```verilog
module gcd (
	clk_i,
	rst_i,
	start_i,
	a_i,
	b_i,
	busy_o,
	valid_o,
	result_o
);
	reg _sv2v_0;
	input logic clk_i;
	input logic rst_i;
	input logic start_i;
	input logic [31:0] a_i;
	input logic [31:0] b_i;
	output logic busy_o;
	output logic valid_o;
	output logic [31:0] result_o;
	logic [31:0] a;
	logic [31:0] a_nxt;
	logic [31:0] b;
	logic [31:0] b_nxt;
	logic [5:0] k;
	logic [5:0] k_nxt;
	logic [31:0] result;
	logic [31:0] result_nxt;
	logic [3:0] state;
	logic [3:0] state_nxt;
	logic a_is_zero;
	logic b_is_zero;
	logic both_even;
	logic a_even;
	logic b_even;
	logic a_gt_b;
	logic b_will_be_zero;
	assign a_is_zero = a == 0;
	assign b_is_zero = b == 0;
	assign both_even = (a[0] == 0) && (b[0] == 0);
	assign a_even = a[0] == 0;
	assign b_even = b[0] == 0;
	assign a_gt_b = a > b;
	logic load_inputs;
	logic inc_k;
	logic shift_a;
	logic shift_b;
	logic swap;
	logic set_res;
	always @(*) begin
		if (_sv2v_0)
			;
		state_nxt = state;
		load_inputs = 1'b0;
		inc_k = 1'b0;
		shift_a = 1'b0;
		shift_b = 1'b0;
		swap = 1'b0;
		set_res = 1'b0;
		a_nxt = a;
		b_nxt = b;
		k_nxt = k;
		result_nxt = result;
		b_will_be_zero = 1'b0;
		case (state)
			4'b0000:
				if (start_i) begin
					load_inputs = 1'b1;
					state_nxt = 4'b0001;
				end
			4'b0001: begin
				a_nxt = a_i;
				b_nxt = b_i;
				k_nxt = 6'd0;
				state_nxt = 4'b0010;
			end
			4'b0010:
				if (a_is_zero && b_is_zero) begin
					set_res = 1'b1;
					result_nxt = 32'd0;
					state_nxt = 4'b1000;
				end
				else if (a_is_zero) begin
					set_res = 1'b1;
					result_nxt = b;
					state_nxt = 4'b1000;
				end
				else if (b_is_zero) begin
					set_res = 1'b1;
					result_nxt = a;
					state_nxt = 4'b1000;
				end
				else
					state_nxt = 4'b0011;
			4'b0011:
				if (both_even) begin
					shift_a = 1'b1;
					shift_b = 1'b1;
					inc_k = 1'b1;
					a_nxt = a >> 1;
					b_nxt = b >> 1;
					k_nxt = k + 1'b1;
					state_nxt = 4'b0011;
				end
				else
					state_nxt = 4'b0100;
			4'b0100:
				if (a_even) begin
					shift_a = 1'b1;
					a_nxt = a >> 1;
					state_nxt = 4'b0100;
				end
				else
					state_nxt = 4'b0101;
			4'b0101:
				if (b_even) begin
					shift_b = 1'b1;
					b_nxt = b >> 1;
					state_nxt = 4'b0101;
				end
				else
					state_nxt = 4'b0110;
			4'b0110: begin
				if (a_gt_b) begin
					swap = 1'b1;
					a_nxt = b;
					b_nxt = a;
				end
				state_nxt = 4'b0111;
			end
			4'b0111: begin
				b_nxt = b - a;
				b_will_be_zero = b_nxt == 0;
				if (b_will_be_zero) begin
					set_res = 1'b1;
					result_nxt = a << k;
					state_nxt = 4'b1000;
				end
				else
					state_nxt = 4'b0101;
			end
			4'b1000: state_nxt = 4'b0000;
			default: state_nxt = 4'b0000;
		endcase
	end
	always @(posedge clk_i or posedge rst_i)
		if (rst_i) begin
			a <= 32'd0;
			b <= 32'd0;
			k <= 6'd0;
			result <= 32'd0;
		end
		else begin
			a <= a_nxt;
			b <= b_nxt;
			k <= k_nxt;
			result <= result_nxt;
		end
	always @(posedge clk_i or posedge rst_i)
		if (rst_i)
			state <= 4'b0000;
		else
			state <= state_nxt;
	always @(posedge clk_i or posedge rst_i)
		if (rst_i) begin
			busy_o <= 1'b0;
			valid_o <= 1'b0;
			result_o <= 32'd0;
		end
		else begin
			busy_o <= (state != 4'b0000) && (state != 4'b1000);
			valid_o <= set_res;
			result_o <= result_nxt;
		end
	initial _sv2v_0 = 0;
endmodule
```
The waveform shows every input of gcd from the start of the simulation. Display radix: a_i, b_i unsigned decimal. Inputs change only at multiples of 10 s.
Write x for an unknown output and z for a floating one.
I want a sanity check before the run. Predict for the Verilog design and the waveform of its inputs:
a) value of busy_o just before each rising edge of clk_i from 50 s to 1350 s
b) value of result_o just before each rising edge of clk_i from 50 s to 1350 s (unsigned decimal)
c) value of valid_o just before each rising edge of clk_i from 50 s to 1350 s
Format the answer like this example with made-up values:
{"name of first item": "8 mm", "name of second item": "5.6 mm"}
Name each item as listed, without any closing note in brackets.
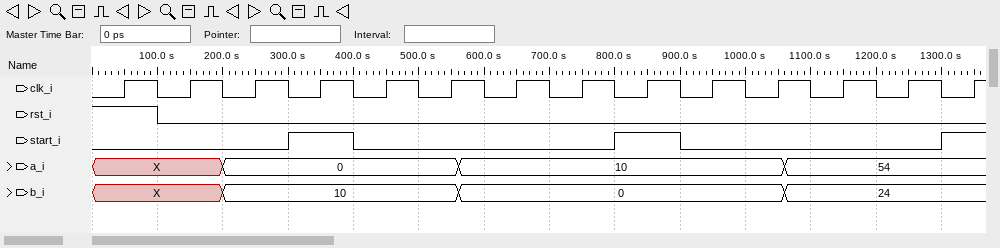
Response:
{"value of busy_o just before each rising edge of clk_i from 50 s to 1350 s": "0 0 0 0 0 1 1 0 0 0 1 1 0 0", "value of result_o just before each rising edge of clk_i from 50 s to 1350 s": "0, 0, 0, 0, 0, 0, 10, 10, 10, 10, 10, 10, 10, 10", "value of valid_o just before each rising edge of clk_i from 50 s to 1350 s": "0 0 0 0 0 0 1 0 0 0 0 1 0 0"}
